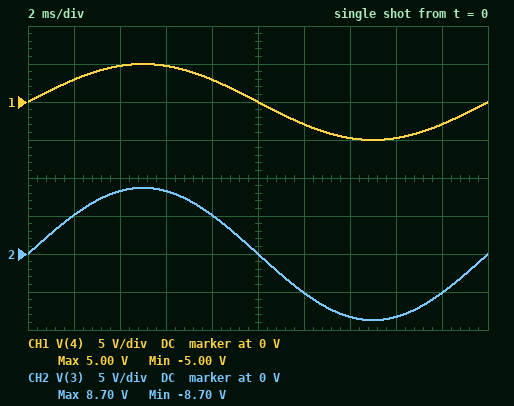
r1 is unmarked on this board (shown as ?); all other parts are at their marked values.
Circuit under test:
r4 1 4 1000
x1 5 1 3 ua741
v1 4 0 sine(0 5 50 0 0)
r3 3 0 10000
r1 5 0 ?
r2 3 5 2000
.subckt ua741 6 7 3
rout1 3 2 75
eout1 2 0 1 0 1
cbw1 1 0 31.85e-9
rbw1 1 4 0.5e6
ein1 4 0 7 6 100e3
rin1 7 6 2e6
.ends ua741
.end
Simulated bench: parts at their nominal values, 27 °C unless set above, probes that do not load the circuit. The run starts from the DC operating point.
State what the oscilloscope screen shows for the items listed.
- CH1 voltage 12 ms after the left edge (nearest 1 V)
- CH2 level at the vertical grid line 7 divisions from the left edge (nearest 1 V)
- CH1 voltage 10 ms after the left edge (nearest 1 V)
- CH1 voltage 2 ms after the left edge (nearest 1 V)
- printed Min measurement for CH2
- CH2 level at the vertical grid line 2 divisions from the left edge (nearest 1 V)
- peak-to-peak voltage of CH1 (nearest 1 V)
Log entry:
-3 V
-8 V
0 V
3 V
-8.70 V
8 V
10 V
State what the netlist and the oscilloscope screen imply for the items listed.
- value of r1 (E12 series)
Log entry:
2.7 kΩ
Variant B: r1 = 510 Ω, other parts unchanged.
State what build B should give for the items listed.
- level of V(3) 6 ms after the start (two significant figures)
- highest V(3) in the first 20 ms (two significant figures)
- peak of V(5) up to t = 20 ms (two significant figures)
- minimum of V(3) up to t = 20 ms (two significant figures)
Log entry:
23 V
25 V
5.0 V
-25 V
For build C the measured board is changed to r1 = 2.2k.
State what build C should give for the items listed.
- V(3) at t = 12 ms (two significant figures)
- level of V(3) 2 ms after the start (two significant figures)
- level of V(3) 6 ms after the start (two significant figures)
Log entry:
-5.6 V
5.6 V
9.1 V
